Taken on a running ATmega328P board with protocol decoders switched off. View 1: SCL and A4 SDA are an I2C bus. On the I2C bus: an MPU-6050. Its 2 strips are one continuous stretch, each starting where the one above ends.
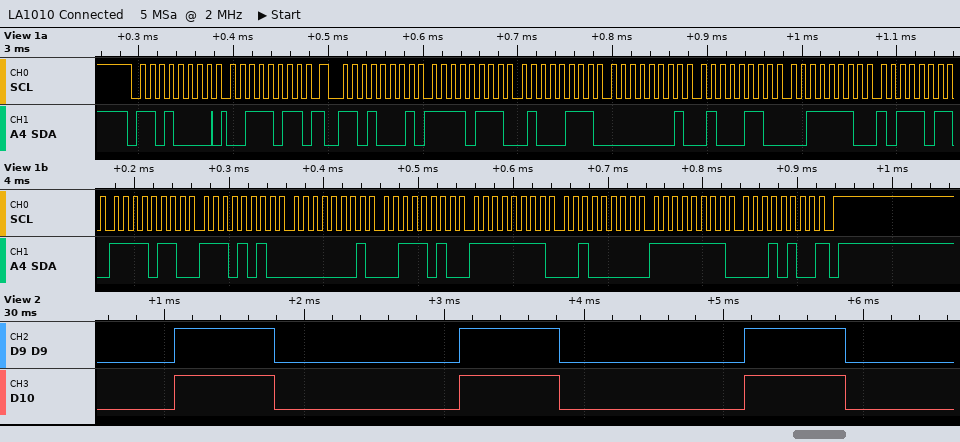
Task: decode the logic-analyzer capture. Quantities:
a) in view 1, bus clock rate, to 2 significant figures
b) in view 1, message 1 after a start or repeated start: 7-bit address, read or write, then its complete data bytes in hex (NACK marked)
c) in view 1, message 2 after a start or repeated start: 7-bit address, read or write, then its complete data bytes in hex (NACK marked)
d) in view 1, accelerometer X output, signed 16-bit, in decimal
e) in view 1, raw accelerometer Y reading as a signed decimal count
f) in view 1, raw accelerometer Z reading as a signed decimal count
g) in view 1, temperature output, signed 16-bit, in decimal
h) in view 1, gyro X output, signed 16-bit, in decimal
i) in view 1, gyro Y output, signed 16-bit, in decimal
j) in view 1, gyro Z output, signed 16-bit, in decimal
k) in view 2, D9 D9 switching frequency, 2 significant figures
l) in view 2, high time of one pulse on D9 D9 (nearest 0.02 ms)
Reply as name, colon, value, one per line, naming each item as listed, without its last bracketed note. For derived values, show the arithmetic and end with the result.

in view 1, bus clock rate, to 2 significant figures: 100 kHz
in view 1, message 1 after a start or repeated start: 7-bit address, read or write, then its complete data bytes in hex: 0x68 write: 3B
in view 1, message 2 after a start or repeated start: 7-bit address, read or write, then its complete data bytes in hex: 0x68 read: F7 47 01 46 3E BB F6 EA 01 3A FF 20 FF 14 NACK
in view 1, accelerometer X output, signed 16-bit, in decimal: 0xF747 = -2233
in view 1, raw accelerometer Y reading as a signed decimal count: 0x0146 = 326
in view 1, raw accelerometer Z reading as a signed decimal count: 0x3EBB = 16059
in view 1, temperature output, signed 16-bit, in decimal: 0xF6EA = -2326
in view 1, gyro X output, signed 16-bit, in decimal: 0x013A = 314
in view 1, gyro Y output, signed 16-bit, in decimal: 0xFF20 = -224
in view 1, gyro Z output, signed 16-bit, in decimal: 0xFF14 = -236
in view 2, D9 D9 switching frequency, 2 significant figures: 490 Hz
in view 2, high time of one pulse on D9 D9: 0.72 ms
